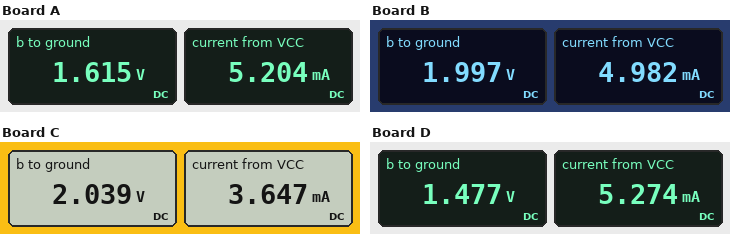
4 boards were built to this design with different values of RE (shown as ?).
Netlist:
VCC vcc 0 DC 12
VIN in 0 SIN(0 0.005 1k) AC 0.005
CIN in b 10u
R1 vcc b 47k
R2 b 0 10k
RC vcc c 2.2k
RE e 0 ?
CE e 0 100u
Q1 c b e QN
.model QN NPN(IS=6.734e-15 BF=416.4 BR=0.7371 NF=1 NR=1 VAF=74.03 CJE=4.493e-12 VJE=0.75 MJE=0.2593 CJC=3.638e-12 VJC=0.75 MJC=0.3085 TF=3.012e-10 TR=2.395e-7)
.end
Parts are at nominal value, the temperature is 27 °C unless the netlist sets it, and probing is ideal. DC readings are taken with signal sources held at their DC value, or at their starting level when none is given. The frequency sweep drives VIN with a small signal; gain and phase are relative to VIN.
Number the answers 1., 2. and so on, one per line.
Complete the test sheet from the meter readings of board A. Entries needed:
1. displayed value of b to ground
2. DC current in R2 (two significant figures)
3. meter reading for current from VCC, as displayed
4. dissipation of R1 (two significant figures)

1. 1.615 V
2. 160 µA
3. 5.204 mA
4. 2.3 mW
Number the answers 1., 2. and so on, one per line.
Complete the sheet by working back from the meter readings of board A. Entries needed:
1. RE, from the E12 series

1. 180 Ω
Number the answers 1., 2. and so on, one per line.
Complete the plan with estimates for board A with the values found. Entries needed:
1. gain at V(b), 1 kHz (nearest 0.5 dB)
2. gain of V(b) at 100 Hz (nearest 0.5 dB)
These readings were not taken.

1. -6.0 dB
2. -18.0 dB
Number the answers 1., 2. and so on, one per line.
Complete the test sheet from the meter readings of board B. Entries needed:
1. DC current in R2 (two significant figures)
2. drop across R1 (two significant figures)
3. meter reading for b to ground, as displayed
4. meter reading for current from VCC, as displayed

1. 200 µA
2. 10 V
3. 1.997 V
4. 4.982 mA
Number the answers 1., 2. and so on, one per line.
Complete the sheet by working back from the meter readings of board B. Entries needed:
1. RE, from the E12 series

1. 270 Ω
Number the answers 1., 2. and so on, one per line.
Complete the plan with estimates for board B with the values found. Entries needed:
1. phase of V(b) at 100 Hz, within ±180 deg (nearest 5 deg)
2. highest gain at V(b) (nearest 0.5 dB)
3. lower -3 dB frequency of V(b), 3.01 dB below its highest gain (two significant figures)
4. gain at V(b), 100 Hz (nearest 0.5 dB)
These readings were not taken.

1. 15 deg
2. 0 dB
3. 410 Hz
4. -6.0 dB
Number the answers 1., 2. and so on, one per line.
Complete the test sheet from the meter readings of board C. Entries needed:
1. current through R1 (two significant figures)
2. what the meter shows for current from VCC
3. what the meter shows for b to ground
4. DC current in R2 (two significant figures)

1. 210 µA
2. 3.647 mA
3. 2.039 V
4. 200 µA
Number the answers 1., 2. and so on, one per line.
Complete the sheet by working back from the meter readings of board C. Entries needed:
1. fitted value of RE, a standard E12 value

1. 390 Ω
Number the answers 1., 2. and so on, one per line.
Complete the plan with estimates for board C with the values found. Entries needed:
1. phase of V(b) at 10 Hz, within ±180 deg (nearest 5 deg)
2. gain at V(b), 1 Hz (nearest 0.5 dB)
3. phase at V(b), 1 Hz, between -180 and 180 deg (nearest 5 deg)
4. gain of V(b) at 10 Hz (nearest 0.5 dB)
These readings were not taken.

1. 10 deg
2. -7.0 dB
3. 65 deg
4. -0.5 dB
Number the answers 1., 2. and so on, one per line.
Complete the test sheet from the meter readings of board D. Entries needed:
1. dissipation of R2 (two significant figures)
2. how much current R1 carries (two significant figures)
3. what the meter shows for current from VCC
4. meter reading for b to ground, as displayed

1. 220 µW
2. 220 µA
3. 5.274 mA
4. 1.477 V
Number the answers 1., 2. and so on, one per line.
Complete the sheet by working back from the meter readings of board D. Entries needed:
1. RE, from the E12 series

1. 150 Ω
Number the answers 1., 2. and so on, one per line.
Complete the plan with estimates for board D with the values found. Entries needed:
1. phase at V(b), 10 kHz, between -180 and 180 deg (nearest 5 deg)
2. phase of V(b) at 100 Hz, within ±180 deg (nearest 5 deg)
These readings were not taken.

1. 10 deg
2. 30 deg
